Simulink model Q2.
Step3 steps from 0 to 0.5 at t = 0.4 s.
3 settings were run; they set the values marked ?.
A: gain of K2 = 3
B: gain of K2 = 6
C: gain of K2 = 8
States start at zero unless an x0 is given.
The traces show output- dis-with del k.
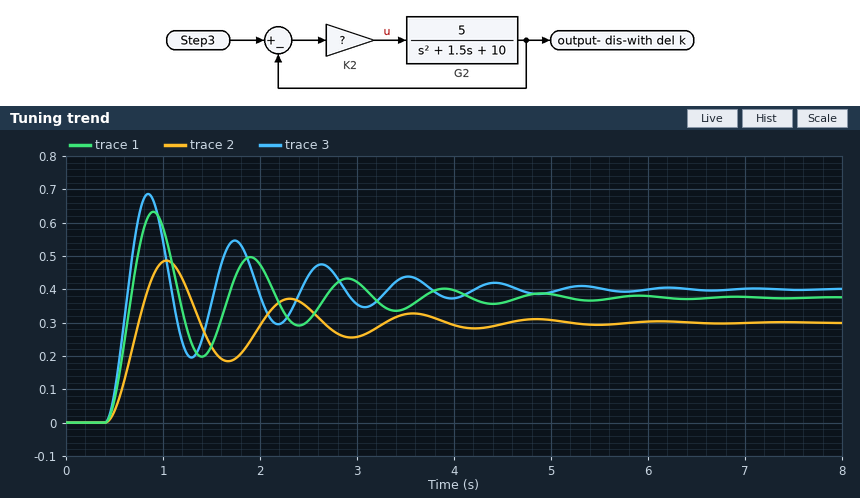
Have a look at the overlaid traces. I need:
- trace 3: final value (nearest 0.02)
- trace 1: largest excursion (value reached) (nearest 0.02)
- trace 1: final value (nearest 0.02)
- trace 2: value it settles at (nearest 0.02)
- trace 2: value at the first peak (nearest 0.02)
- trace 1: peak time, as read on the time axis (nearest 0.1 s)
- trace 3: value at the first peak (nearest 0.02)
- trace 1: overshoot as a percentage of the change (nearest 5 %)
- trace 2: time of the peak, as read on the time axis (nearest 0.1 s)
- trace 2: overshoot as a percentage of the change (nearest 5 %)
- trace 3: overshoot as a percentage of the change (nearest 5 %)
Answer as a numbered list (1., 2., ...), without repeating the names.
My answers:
1. 0.40
2. 0.64
3. 0.38
4. 0.30
5. 0.48
6. 0.9 s
7. 0.68
8. 70 %
9. 1.0 s
10. 60 %
11. 70 %
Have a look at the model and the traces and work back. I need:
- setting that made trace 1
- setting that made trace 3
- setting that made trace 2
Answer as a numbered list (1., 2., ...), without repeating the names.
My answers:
1. B
2. C
3. A
